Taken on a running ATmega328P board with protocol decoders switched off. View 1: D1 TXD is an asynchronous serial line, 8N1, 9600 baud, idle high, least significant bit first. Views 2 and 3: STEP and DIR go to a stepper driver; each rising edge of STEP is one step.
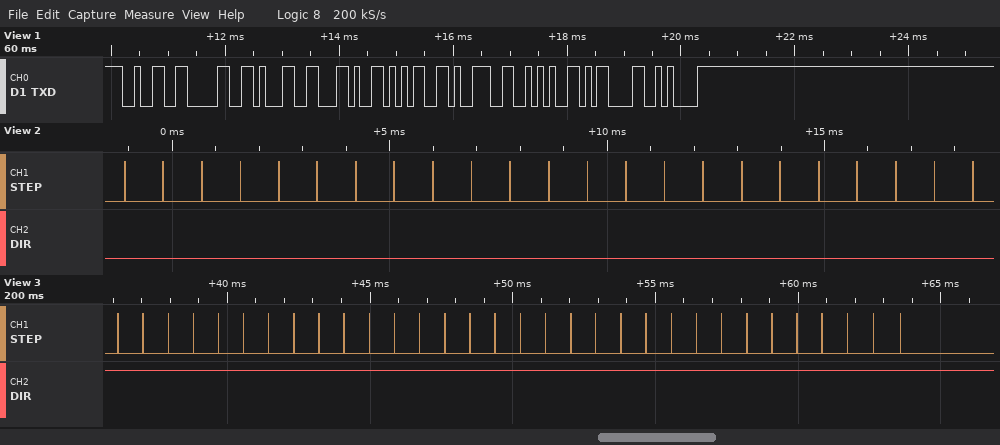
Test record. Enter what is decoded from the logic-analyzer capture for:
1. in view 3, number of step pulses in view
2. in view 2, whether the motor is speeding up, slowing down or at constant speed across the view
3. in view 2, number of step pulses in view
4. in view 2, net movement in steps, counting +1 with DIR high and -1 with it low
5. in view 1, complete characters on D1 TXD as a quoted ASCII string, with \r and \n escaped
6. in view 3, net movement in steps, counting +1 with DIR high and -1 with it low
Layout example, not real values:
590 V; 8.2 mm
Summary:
32; constant speed; 23; -23; "201,59*\r\n"; +32
